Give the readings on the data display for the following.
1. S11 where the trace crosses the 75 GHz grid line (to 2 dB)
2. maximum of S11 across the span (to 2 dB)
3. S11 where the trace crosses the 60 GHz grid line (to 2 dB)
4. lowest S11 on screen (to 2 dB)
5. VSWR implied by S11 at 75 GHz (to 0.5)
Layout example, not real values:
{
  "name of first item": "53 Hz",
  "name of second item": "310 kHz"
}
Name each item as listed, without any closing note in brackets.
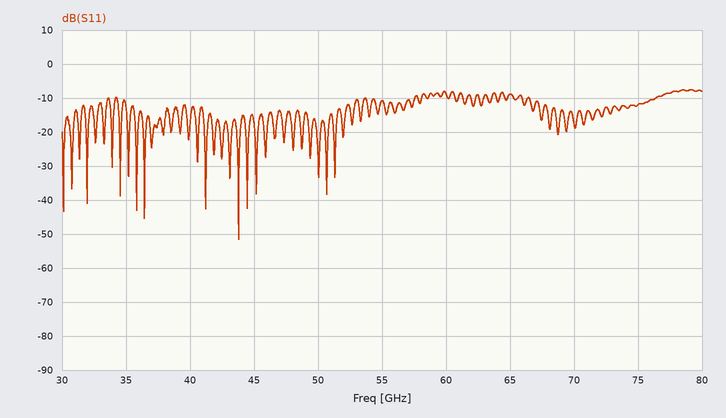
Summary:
{
  "S11 where the trace crosses the 75 GHz grid line": "-12 dB",
  "maximum of S11 across the span": "-8 dB",
  "S11 where the trace crosses the 60 GHz grid line": "-8 dB",
  "lowest S11 on screen": "-52 dB",
  "VSWR implied by S11 at 75 GHz": "1.5"
}
